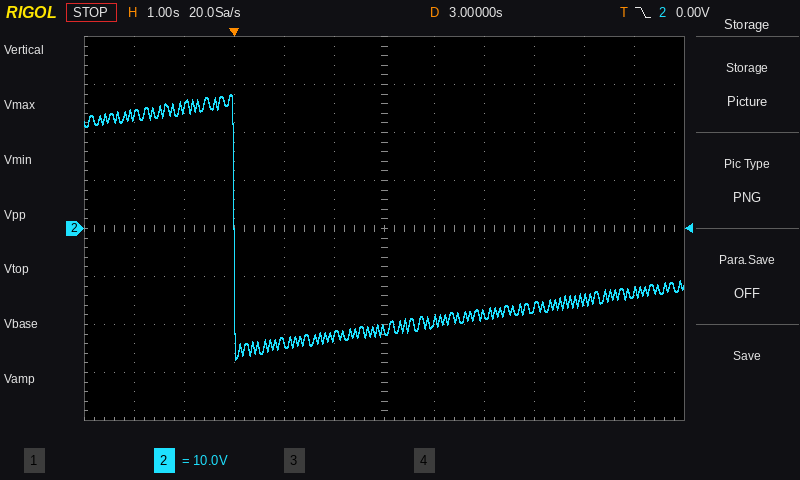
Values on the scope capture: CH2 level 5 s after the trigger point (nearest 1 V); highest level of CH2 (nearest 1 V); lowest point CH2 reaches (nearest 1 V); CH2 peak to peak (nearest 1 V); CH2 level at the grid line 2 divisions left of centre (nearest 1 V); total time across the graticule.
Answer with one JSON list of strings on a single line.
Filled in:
["-18 V", "28 V", "-27 V", "55 V", "-24 V", "12 s"]
